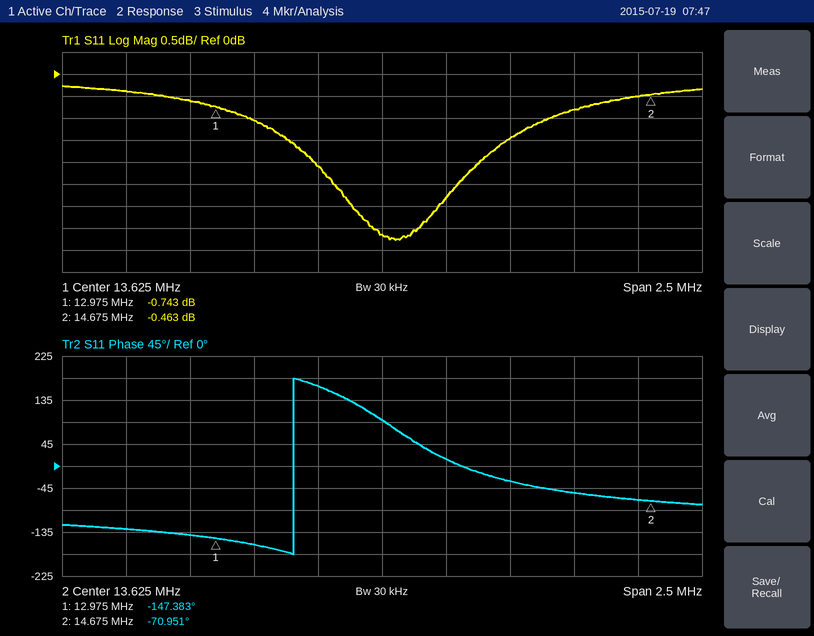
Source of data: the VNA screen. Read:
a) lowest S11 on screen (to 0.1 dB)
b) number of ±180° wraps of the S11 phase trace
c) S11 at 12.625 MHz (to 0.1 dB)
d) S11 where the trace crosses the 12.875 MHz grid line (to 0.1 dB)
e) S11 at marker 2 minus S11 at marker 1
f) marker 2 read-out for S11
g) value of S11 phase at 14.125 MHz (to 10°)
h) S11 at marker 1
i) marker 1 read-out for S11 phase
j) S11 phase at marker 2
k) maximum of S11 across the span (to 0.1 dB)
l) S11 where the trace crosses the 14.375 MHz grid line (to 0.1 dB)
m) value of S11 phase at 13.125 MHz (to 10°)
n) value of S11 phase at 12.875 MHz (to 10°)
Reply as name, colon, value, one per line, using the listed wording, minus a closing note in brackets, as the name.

lowest S11 on screen: -3.8 dB
number of ±180° wraps of the S11 phase trace: 1
S11 at 12.625 MHz: -0.4 dB
S11 where the trace crosses the 12.875 MHz grid line: -0.6 dB
S11 at marker 2 minus S11 at marker 1: 0.280 dB
marker 2 read-out for S11: -0.463 dB
value of S11 phase at 14.125 MHz: -30°
S11 at marker 1: -0.743 dB
marker 1 read-out for S11 phase: -147.383°
S11 phase at marker 2: -70.951°
maximum of S11 across the span: -0.3 dB
S11 where the trace crosses the 14.375 MHz grid line: -0.8 dB
value of S11 phase at 13.125 MHz: -160°
value of S11 phase at 12.875 MHz: -140°
